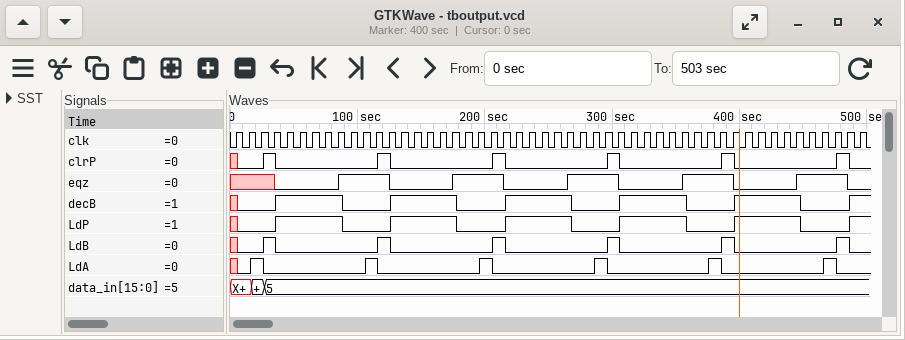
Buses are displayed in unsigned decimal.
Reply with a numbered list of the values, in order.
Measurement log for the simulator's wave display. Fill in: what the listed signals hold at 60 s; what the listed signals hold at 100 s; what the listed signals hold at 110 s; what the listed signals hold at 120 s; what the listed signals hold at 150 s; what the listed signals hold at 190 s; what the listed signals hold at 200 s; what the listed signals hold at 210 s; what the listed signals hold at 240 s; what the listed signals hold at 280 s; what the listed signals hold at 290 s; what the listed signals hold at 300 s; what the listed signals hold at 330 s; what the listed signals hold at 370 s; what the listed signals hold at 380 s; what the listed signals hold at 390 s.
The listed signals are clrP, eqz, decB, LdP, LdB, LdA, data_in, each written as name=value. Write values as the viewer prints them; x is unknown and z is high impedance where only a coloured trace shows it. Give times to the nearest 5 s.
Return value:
1. clrP=0, eqz=0, decB=1, LdP=1, LdB=0, LdA=0, data_in=5
2. clrP=0, eqz=1, decB=0, LdP=0, LdB=0, LdA=0, data_in=5
3. clrP=0, eqz=1, decB=0, LdP=0, LdB=0, LdA=1, data_in=5
4. clrP=1, eqz=1, decB=0, LdP=0, LdB=1, LdA=0, data_in=5
5. clrP=0, eqz=0, decB=1, LdP=1, LdB=0, LdA=0, data_in=5
6. clrP=0, eqz=1, decB=0, LdP=0, LdB=0, LdA=0, data_in=5
7. clrP=0, eqz=1, decB=0, LdP=0, LdB=0, LdA=1, data_in=5
8. clrP=1, eqz=1, decB=0, LdP=0, LdB=1, LdA=0, data_in=5
9. clrP=0, eqz=0, decB=1, LdP=1, LdB=0, LdA=0, data_in=5
10. clrP=0, eqz=1, decB=0, LdP=0, LdB=0, LdA=0, data_in=5
11. clrP=0, eqz=1, decB=0, LdP=0, LdB=0, LdA=1, data_in=5
12. clrP=1, eqz=1, decB=0, LdP=0, LdB=1, LdA=0, data_in=5
13. clrP=0, eqz=0, decB=1, LdP=1, LdB=0, LdA=0, data_in=5
14. clrP=0, eqz=1, decB=0, LdP=0, LdB=0, LdA=0, data_in=5
15. clrP=0, eqz=1, decB=0, LdP=0, LdB=0, LdA=1, data_in=5
16. clrP=1, eqz=1, decB=0, LdP=0, LdB=1, LdA=0, data_in=5
